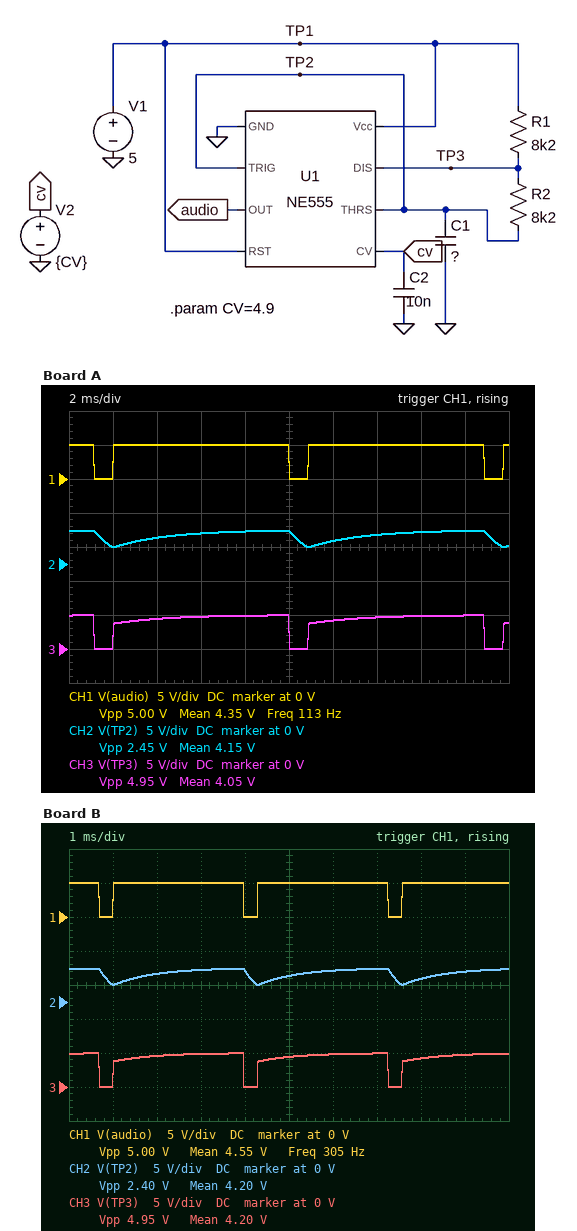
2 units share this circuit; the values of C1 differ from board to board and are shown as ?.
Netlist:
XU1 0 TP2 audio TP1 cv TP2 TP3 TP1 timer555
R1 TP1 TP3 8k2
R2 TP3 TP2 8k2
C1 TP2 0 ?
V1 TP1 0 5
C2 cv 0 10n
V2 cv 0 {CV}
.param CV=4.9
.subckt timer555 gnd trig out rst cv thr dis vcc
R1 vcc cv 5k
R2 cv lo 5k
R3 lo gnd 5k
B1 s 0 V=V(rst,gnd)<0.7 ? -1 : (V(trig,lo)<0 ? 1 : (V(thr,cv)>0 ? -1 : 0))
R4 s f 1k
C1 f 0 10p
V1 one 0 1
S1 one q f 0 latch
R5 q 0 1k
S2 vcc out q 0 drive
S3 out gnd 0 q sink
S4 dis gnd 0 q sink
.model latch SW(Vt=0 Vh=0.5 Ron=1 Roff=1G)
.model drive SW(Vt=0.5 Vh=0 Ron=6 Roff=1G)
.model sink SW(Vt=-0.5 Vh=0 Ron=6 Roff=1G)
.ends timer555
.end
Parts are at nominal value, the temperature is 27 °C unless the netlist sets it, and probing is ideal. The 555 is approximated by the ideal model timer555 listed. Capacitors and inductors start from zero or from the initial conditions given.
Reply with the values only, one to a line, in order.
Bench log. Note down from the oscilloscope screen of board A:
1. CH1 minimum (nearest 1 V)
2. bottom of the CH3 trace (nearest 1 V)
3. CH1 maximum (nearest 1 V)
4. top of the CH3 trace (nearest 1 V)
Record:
0 V
0 V
5 V
5 V
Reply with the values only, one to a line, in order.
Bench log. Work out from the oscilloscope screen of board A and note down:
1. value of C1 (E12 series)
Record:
150 nF
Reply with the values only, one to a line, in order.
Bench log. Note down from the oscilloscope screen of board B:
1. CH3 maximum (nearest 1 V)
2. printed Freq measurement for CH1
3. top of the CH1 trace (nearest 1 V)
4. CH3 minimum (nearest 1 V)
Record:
5 V
305 Hz
5 V
0 V
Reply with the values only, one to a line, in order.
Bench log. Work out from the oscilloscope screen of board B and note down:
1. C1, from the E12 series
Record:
56 nF
